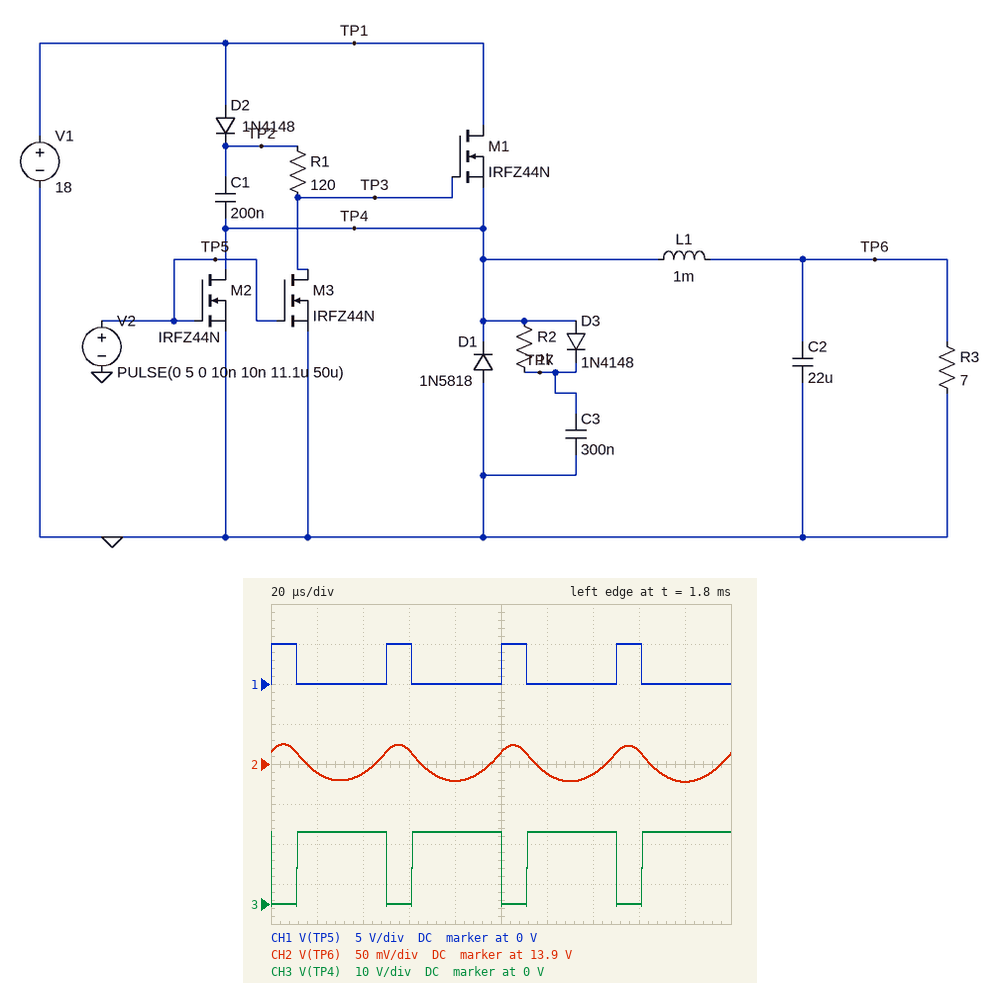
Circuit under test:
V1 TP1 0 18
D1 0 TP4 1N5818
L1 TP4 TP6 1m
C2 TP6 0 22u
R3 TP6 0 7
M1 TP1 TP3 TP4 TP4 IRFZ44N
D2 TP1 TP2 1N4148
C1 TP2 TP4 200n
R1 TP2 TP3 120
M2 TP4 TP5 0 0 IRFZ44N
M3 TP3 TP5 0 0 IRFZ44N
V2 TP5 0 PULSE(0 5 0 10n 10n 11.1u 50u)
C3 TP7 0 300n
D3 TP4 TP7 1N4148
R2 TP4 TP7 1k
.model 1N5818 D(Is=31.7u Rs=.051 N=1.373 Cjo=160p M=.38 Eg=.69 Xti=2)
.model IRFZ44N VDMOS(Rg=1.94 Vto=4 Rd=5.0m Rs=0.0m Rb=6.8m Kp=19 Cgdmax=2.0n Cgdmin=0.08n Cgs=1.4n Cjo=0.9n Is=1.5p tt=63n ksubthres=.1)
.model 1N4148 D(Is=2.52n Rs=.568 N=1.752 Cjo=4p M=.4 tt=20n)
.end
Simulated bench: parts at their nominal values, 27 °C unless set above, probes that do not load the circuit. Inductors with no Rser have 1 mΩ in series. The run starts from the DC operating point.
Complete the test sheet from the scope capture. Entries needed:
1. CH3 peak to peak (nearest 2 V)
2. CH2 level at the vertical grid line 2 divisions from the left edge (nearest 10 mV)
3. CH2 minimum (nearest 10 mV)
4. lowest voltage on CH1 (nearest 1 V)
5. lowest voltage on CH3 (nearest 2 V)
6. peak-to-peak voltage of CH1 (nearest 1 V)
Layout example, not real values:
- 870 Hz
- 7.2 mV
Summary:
- 18 V
- 13.89 V
- 13.88 V
- 0 V
- 0 V
- 5 V
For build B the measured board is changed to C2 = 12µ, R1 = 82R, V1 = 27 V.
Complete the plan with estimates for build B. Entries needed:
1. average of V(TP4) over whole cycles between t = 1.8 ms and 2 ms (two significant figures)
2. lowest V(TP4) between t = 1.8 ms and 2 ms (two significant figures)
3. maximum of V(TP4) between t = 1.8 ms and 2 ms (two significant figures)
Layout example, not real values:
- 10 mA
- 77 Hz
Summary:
- 21 V
- -560 mV
- 27 V
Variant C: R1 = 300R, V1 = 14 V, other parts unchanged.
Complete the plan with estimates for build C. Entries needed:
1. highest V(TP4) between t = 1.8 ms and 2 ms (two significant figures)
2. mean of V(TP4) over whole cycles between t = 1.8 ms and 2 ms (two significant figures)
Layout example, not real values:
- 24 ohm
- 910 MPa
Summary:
- 14 V
- 11 V
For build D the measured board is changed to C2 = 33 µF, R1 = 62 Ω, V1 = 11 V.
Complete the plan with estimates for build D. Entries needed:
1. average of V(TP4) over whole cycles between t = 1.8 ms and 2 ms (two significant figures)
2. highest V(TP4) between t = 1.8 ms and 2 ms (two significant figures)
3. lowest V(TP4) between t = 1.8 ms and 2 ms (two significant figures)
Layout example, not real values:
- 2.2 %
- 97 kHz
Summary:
- 8.5 V
- 11 V
- -450 mV
